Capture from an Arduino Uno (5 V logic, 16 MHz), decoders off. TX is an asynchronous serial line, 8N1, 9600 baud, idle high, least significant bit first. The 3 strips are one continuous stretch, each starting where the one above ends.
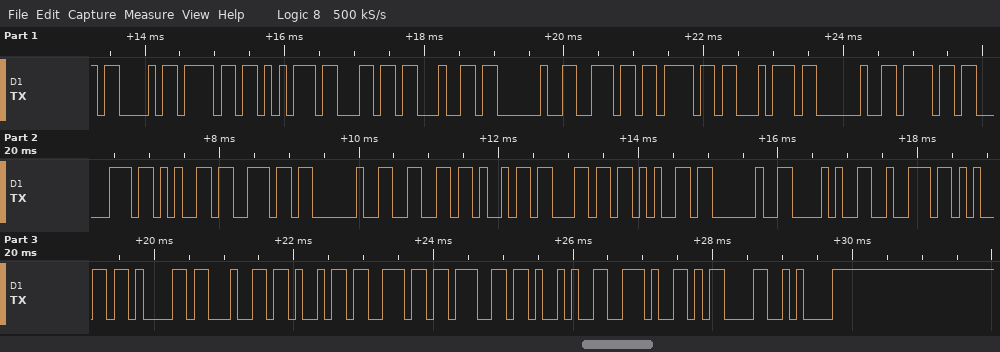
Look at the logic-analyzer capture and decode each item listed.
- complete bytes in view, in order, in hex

43 6F 75 6C 64 20 6E 6F 74 20 6F 70 65 6E 20 66 69 6C 65 20 28 72 65 61 64 69 6E 67 29 2E 0D 0A
